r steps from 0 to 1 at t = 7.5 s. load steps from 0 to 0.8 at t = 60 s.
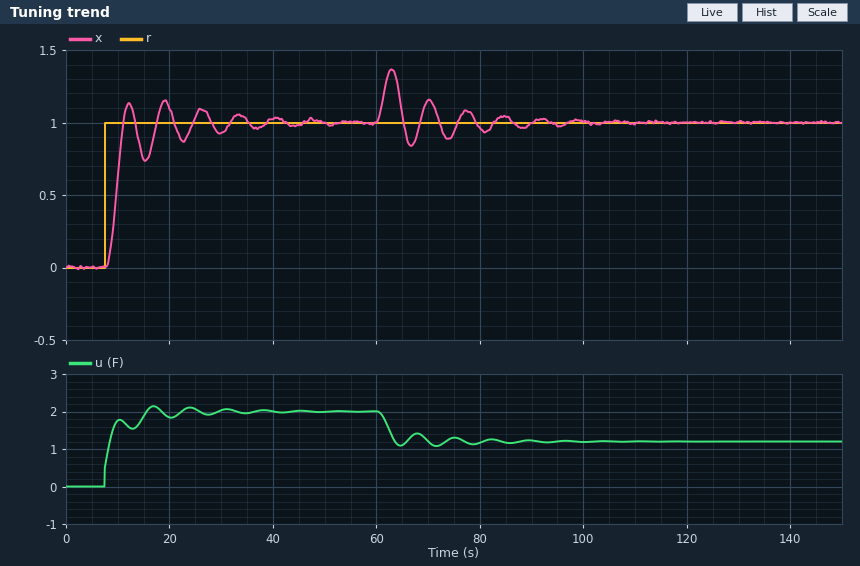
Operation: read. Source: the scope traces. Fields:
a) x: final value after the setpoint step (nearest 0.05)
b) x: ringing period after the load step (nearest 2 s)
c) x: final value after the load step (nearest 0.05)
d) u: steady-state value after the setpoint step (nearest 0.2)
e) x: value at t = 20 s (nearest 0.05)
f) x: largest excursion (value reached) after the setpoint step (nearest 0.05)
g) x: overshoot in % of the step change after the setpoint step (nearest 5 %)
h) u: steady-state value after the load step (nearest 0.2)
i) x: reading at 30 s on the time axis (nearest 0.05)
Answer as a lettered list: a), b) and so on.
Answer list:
a) 1.00
b) 8 s
c) 1.00
d) 2.0
e) 1.10
f) 1.15
g) 15 %
h) 1.2
i) 0.95
